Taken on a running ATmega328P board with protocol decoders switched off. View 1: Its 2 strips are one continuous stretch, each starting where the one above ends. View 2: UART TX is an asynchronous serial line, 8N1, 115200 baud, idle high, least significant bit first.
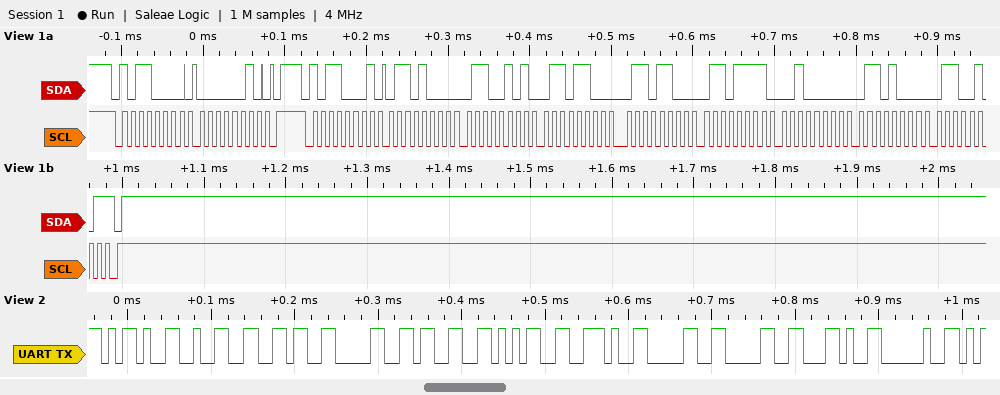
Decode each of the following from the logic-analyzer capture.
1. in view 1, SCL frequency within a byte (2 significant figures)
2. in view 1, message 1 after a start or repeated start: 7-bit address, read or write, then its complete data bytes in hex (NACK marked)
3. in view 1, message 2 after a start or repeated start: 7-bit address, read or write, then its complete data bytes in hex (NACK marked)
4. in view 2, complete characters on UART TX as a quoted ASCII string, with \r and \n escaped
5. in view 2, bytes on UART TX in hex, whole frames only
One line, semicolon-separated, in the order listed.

100 kHz; 0x58 write: 02; 0x58 read: 68 65 6C 6C 6F 20 68 65 NACK; "-26035.00, "; 0x2D 0x32 0x36 0x30 0x33 0x35 0x2E 0x30 0x30 0x2C 0x20
